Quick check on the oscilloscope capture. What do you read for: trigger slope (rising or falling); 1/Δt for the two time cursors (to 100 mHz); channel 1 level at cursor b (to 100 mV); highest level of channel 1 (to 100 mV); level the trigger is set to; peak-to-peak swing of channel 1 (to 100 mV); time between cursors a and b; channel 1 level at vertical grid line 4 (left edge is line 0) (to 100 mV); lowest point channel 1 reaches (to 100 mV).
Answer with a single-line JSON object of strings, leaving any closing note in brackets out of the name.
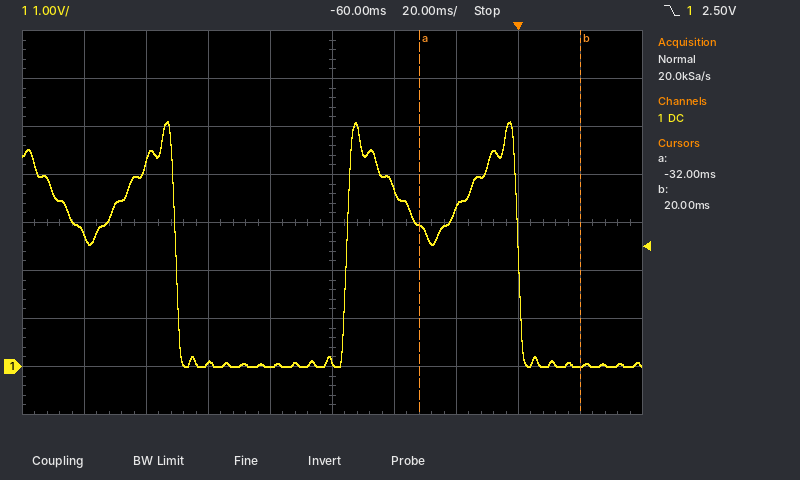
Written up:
{"trigger slope": "falling", "1/Δt for the two time cursors": "19.2 Hz", "channel 1 level at cursor b": "0.0 V", "highest level of channel 1": "5.1 V", "level the trigger is set to": "2.50 V", "peak-to-peak swing of channel 1": "5.1 V", "time between cursors a and b": "52 ms", "channel 1 level at vertical grid line 4 (left edge is line 0)": "0.0 V", "lowest point channel 1 reaches": "0.0 V"}
